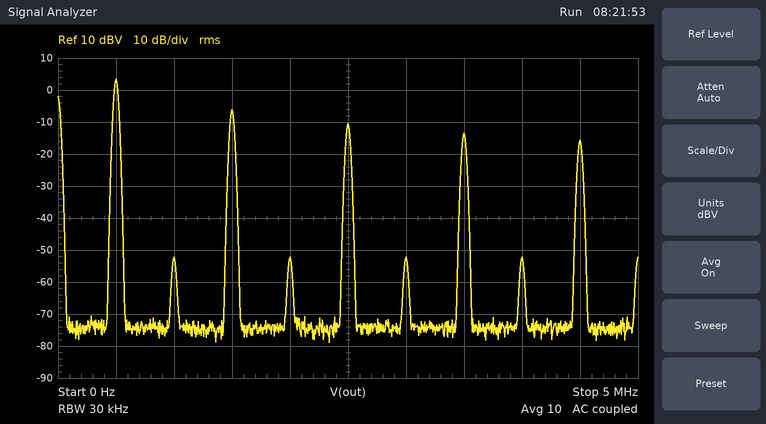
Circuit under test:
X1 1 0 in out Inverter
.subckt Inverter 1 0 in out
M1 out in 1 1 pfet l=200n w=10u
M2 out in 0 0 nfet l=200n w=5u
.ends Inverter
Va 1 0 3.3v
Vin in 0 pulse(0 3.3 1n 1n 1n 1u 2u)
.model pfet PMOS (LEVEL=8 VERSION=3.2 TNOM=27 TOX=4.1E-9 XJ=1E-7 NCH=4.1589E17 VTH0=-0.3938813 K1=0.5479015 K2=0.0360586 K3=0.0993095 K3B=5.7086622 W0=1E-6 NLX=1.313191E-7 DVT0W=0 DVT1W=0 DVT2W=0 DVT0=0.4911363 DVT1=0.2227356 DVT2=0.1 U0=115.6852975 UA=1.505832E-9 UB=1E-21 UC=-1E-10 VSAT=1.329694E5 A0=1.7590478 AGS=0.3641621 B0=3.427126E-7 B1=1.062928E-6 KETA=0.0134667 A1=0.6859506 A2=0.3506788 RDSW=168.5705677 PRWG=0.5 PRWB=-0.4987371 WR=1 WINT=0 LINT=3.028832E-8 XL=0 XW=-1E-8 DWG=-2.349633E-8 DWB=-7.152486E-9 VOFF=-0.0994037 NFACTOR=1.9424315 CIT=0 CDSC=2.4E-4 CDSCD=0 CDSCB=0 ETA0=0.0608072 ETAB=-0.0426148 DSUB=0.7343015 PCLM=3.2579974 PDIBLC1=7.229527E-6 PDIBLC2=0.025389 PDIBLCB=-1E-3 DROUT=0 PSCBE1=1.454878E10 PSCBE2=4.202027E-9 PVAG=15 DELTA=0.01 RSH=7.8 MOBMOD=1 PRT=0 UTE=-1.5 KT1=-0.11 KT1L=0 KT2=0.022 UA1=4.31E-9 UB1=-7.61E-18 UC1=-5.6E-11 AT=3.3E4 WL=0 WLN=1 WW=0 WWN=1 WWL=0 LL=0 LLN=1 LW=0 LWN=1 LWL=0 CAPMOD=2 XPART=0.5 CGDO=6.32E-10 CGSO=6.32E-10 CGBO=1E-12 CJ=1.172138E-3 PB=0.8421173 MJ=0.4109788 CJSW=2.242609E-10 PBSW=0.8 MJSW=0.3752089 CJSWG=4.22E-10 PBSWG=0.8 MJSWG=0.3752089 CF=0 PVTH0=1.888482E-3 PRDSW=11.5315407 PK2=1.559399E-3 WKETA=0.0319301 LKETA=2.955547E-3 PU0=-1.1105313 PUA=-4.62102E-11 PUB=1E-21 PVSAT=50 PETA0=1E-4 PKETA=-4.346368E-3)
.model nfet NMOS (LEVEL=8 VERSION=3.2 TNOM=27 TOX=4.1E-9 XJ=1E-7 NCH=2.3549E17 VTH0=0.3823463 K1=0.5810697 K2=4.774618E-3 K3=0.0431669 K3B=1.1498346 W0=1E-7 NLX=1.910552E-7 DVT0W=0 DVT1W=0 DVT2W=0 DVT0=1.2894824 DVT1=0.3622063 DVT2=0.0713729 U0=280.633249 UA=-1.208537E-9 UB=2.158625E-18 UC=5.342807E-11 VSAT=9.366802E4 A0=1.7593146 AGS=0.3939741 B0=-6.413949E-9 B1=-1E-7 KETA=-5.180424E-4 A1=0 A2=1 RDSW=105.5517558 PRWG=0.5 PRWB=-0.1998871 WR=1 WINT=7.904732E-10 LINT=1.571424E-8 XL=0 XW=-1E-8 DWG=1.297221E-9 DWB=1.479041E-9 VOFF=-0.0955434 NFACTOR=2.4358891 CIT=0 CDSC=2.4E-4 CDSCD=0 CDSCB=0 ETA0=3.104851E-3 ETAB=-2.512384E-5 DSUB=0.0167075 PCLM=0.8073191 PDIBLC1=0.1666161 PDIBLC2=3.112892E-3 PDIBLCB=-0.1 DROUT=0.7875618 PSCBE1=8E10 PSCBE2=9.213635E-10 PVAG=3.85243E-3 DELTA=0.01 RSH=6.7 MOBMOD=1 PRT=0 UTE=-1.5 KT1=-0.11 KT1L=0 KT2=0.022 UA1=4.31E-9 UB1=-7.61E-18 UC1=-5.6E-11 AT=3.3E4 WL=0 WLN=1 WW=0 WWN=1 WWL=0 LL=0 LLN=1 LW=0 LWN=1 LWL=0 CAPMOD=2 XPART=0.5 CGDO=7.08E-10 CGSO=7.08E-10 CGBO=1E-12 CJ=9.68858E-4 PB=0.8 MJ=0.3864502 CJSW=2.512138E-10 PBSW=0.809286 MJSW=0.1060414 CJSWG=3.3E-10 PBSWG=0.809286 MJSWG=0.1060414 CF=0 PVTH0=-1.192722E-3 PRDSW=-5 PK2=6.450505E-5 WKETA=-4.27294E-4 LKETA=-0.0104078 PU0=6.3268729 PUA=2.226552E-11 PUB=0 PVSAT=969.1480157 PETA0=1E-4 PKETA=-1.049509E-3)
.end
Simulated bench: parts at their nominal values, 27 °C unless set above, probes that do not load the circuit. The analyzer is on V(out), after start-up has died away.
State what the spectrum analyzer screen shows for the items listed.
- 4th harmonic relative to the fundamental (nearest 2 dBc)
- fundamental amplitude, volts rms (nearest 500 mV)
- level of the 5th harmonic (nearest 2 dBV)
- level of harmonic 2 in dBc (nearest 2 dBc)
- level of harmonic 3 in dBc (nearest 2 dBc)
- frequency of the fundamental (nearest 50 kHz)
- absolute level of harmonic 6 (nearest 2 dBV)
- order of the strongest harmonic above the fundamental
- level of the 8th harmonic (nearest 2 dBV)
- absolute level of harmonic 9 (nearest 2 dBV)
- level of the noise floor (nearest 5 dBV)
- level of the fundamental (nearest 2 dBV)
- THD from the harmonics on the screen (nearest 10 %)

-56 dBc
1.5 V
-10 dBV
-56 dBc
-10 dBc
500 kHz
-52 dBV
3
-52 dBV
-16 dBV
-75 dBV
4 dBV
40 %
